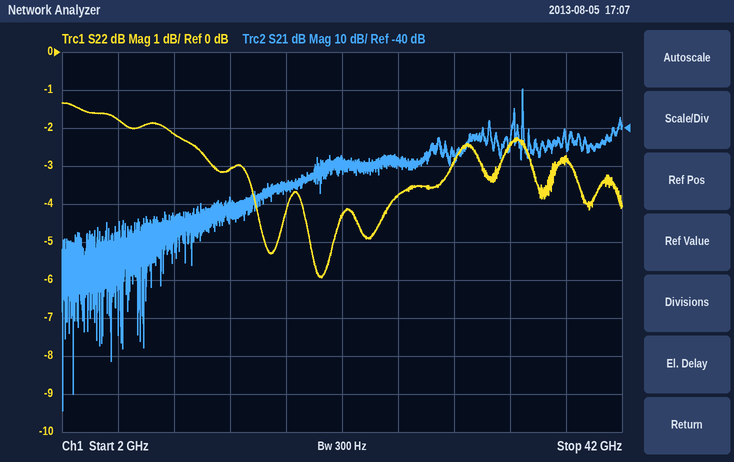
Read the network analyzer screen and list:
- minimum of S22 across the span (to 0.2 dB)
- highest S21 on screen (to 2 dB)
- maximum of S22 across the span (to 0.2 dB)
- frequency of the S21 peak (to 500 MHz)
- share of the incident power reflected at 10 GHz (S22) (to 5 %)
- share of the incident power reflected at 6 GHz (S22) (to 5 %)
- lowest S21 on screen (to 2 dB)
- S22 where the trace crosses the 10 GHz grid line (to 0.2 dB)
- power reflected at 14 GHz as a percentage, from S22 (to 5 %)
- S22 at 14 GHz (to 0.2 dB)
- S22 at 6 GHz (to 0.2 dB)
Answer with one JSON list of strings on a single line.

["-6.0 dB", "-30 dB", "-1.4 dB", "35.0 GHz", "60 %", "65 %", "-114 dB", "-2.2 dB", "50 %", "-3.0 dB", "-1.8 dB"]
